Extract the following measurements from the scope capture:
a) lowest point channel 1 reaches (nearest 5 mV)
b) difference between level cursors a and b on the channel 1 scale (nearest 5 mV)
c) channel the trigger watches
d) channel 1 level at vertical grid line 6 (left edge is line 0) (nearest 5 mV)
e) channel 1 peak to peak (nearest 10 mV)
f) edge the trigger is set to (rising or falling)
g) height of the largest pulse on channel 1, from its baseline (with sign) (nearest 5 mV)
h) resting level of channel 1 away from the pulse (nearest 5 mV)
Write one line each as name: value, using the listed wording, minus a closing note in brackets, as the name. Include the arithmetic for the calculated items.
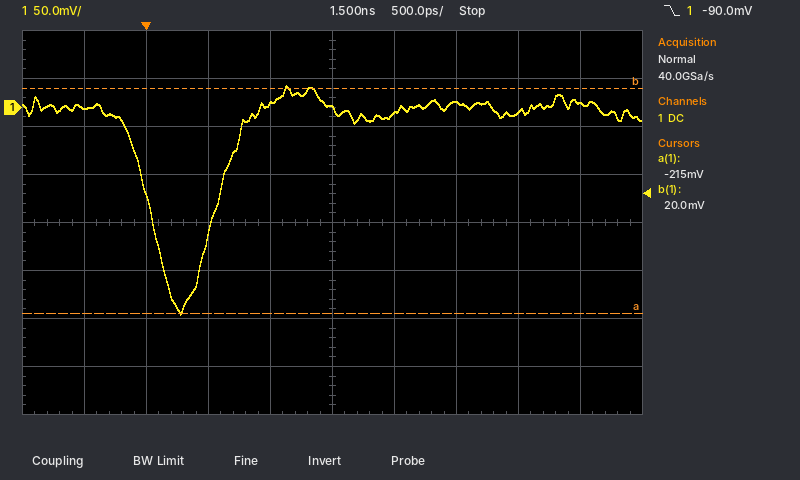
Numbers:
lowest point channel 1 reaches: -215 mV
difference between level cursors a and b on the channel 1 scale: 235 mV
channel the trigger watches: channel 1
channel 1 level at vertical grid line 6 (left edge is line 0): -5 mV
channel 1 peak to peak: 240 mV
edge the trigger is set to: falling
height of the largest pulse on channel 1, from its baseline (with sign): -215 mV − (0 mV) = -215 mV
resting level of channel 1 away from the pulse: 0 mV
